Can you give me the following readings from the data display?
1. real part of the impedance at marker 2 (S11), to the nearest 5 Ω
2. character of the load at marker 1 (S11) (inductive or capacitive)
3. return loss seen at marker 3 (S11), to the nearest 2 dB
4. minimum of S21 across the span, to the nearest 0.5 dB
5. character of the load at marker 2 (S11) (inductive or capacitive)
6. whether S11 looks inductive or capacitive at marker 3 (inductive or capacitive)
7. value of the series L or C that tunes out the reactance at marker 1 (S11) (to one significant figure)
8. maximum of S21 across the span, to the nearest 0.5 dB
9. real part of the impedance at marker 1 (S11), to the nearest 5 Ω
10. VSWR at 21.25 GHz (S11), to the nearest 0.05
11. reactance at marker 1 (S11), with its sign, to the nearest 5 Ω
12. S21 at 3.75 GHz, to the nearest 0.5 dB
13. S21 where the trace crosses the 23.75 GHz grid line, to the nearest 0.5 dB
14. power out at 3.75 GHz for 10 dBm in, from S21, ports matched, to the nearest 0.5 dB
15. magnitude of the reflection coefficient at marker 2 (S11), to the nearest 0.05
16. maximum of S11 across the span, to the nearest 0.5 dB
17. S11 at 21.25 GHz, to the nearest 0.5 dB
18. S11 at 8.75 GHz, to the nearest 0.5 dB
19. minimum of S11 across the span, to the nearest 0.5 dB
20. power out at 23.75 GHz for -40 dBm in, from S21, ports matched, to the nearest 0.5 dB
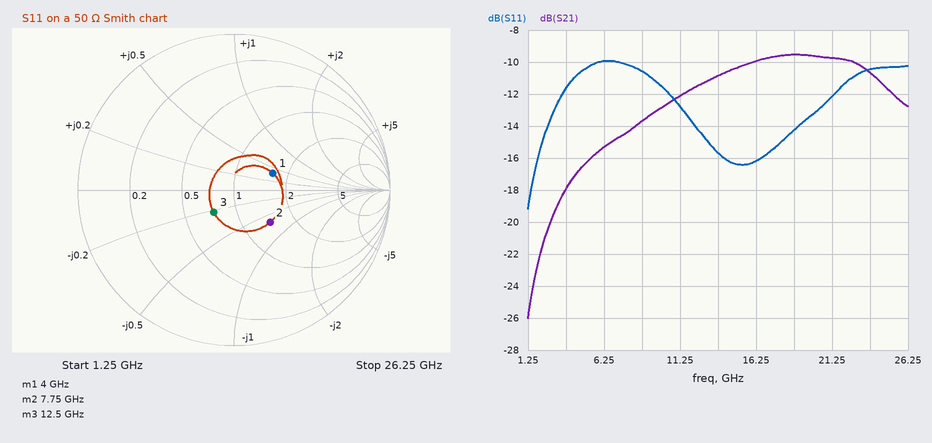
70 Ω
inductive
14 dB
-26.0 dB
capacitive
capacitive
2 pF
-9.5 dB
80 Ω
1.65
+20 Ω
-18.0 dB
-10.5 dB
-8.0 dBm
0.30
-10.0 dB
-12.0 dB
-10.5 dB
-19.0 dB
-50.5 dBm
